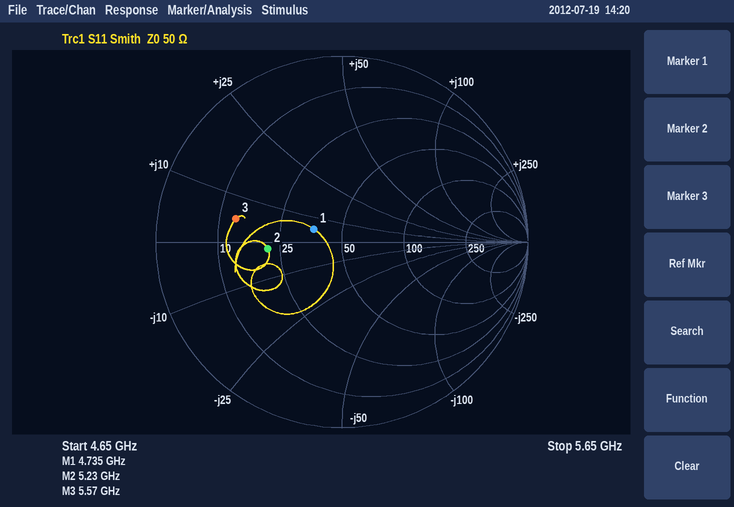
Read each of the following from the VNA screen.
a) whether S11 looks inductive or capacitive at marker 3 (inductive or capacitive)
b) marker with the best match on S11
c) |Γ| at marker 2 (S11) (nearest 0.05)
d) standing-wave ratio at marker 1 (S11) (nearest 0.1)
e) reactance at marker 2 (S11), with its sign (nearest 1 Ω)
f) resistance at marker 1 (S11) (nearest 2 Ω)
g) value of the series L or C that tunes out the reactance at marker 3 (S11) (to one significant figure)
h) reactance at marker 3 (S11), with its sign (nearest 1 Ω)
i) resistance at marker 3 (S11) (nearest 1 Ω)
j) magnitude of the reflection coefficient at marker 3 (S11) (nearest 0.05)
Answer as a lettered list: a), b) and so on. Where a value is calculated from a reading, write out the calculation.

a) inductive
b) marker 1
c) 0.40
d) 1.4
e) -2 Ω
f) 36 Ω
g) C = 1/(2π × 5.57 GHz × 5 Ω) ≈ 6 pF
h) +5 Ω
i) 13 Ω
j) 0.60
